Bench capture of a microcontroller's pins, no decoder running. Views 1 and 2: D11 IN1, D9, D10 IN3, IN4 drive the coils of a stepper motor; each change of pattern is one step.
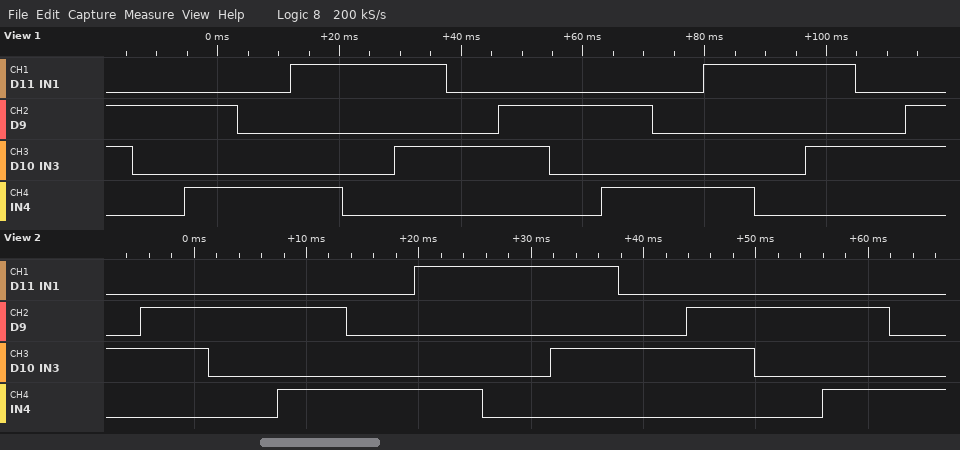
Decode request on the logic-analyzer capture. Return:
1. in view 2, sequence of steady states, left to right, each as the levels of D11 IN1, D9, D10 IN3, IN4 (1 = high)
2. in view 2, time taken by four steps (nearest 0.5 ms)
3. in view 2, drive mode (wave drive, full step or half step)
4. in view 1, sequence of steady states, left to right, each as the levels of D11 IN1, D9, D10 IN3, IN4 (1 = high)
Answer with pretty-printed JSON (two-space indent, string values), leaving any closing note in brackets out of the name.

{
  "in view 2, sequence of steady states, left to right, each as the levels of D11 IN1, D9, D10 IN3, IN4": "0010 0110 0100 0101 0001 1001 1000 1010 0010 0110 0100 0101 0001",
  "in view 2, time taken by four steps": "24.5 ms",
  "in view 2, drive mode": "half step",
  "in view 1, sequence of steady states, left to right, each as the levels of D11 IN1, D9, D10 IN3, IN4": "0110 0100 0101 0001 1001 1000 1010 0010 0110 0100 0101 0001 1001 1000 1010 0010 0110"
}
